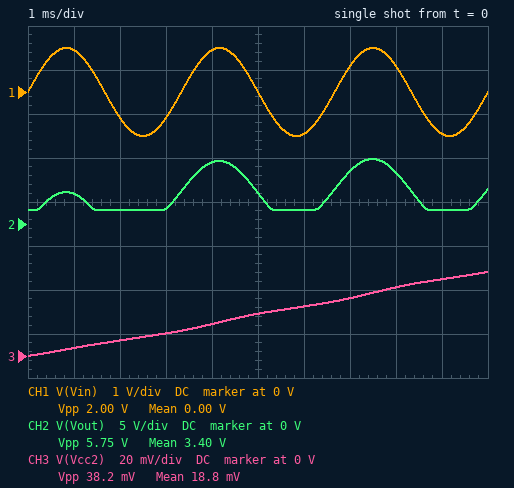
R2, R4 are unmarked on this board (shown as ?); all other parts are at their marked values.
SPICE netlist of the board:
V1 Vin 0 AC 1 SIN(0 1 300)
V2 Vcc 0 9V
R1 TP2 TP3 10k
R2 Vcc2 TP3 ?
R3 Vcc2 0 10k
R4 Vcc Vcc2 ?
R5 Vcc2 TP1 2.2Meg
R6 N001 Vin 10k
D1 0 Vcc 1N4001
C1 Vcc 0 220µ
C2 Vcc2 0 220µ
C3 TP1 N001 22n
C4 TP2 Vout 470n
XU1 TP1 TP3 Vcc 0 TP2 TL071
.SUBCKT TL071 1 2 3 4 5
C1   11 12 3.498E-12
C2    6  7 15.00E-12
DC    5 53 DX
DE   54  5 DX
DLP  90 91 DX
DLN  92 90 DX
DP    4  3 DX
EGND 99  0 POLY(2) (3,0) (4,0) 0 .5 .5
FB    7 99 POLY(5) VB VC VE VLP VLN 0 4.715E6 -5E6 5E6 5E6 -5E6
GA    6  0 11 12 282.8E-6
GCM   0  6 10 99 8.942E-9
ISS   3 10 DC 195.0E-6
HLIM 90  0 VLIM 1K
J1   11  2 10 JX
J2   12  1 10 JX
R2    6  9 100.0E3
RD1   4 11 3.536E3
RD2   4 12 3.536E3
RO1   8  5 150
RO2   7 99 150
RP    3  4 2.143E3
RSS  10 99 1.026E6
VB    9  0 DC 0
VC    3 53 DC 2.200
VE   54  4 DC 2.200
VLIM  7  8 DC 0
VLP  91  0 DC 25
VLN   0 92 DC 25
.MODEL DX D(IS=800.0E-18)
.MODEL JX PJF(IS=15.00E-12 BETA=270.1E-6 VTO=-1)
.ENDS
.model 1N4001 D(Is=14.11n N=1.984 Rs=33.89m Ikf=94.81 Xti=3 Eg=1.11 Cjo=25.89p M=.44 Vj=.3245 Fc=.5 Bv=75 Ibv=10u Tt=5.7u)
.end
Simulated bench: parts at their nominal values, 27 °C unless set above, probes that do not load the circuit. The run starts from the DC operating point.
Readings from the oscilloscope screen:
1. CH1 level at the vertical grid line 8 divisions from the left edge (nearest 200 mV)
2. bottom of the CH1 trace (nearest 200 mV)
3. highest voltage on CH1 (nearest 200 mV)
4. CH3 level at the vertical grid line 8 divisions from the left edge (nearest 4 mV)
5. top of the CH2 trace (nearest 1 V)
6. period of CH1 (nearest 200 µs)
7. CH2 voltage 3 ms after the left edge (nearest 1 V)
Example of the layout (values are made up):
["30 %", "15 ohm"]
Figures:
["600 mV", "-1.0 V", "1.0 V", "32 mV", "7 V", "3.4 ms", "2 V"]
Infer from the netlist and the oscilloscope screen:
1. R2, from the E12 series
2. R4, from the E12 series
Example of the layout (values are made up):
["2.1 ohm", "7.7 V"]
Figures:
["3.9 kΩ", "15 kΩ"]
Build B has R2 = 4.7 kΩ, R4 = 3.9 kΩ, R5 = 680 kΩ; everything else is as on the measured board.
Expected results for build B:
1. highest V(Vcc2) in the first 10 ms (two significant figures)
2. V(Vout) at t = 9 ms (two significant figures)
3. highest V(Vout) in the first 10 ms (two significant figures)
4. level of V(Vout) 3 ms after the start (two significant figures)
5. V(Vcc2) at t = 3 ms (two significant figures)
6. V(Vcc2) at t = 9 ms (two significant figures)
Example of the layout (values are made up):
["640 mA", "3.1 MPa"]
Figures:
["110 mV", "1.6 V", "6.0 V", "1.6 V", "33 mV", "100 mV"]
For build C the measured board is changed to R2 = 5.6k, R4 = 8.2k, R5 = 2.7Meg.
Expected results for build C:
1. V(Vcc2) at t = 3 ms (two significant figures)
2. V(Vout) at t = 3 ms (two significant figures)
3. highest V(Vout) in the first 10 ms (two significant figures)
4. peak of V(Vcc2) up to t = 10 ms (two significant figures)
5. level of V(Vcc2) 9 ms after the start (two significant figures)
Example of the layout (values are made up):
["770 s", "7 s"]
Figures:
["17 mV", "1.6 V", "5.8 V", "58 mV", "52 mV"]
